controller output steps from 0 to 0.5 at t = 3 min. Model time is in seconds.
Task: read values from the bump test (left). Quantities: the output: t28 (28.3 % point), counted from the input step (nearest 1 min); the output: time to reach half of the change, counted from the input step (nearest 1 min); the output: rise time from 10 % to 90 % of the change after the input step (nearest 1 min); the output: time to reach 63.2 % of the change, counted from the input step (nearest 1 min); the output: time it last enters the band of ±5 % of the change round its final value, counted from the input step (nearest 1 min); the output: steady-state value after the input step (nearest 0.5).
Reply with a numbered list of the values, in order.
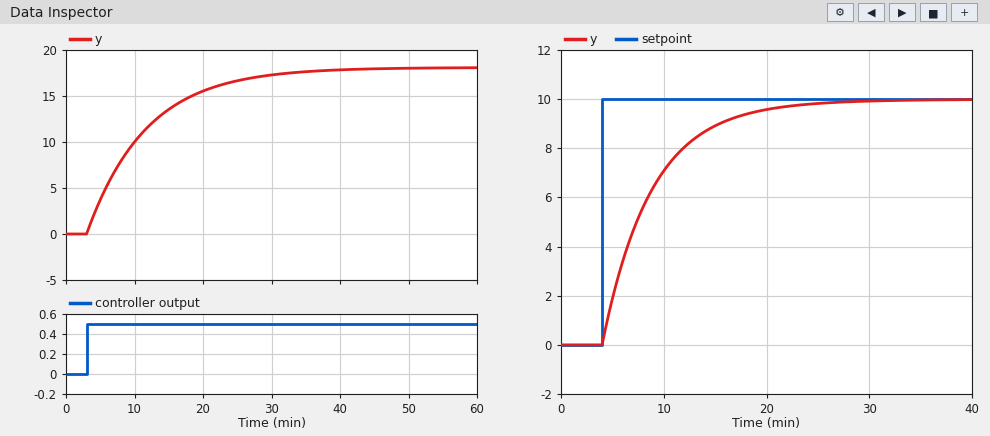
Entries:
1. 3 min
2. 6 min
3. 19 min
4. 9 min
5. 26 min
6. 18.0
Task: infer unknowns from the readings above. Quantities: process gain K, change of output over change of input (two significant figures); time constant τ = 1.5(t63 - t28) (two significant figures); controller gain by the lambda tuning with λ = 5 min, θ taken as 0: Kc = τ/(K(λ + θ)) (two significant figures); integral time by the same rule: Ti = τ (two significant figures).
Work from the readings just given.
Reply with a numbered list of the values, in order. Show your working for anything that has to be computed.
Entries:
1. (18 - 0) / 0.5 = 36
2. 1.5 × (9 - 3) = 9.0 min
3. 9 / (36 × (5 + 0)) = 0.050
4. 9.0 min
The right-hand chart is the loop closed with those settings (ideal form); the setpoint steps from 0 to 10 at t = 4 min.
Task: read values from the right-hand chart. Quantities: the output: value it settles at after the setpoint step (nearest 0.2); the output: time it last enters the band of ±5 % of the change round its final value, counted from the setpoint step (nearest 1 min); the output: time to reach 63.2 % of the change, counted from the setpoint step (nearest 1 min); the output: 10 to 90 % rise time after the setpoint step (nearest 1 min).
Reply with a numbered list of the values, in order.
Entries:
1. 10.0
2. 15 min
3. 5 min
4. 11 min
